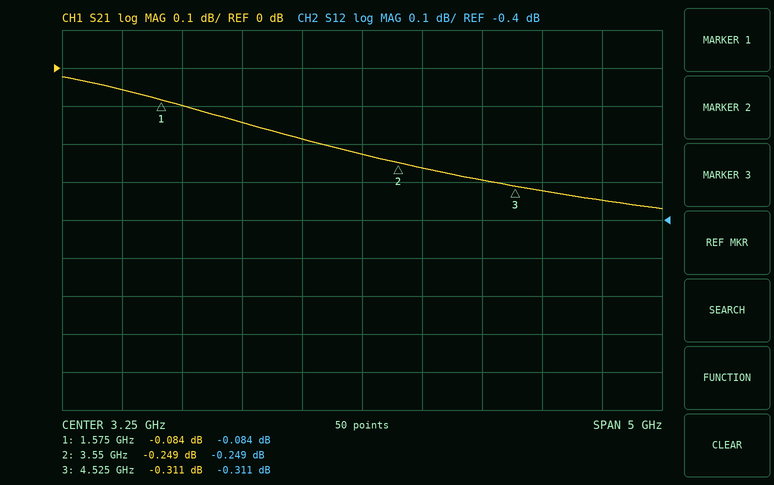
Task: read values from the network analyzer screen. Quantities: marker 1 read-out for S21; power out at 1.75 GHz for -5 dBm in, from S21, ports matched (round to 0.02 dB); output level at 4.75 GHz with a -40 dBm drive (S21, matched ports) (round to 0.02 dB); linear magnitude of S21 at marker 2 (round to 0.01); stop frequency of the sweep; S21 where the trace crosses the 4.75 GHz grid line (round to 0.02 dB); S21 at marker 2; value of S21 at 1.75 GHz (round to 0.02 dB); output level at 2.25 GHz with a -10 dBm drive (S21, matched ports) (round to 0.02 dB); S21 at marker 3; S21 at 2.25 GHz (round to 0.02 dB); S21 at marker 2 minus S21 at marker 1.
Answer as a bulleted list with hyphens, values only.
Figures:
- -0.084 dB
- -5.10 dBm
- -40.32 dBm
- 0.97
- 5.75 GHz
- -0.32 dB
- -0.249 dB
- -0.10 dB
- -10.14 dBm
- -0.311 dB
- -0.14 dB
- -0.165 dB
